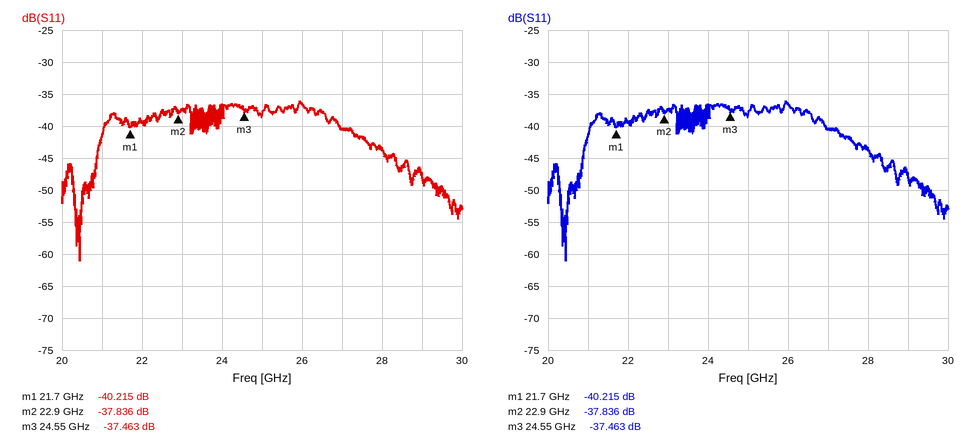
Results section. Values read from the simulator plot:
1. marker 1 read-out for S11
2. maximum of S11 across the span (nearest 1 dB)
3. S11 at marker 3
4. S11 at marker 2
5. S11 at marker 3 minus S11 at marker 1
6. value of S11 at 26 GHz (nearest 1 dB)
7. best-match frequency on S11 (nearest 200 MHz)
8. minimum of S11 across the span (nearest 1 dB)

-40.215 dB
-36 dB
-37.463 dB
-37.836 dB
2.752 dB
-37 dB
20.4 GHz
-61 dB
